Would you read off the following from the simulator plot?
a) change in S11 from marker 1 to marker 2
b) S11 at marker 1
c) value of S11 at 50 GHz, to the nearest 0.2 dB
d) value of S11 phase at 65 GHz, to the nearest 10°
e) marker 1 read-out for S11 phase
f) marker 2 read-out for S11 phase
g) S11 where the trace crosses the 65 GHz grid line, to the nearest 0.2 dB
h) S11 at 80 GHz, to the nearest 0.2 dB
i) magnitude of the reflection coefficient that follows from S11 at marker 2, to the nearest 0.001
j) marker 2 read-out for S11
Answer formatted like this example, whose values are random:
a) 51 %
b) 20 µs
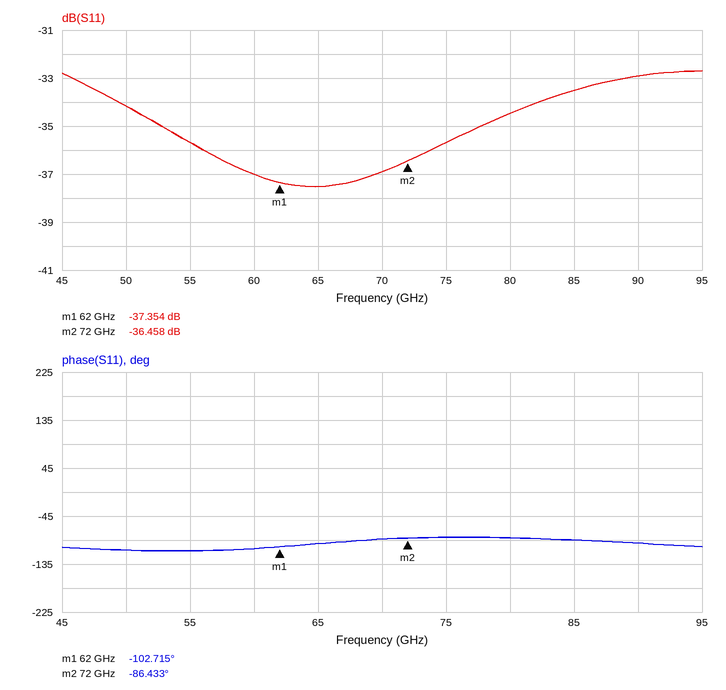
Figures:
a) 0.896 dB
b) -37.354 dB
c) -34.2 dB
d) -100°
e) -102.715°
f) -86.433°
g) -37.6 dB
h) -34.4 dB
i) 0.015
j) -36.458 dB
